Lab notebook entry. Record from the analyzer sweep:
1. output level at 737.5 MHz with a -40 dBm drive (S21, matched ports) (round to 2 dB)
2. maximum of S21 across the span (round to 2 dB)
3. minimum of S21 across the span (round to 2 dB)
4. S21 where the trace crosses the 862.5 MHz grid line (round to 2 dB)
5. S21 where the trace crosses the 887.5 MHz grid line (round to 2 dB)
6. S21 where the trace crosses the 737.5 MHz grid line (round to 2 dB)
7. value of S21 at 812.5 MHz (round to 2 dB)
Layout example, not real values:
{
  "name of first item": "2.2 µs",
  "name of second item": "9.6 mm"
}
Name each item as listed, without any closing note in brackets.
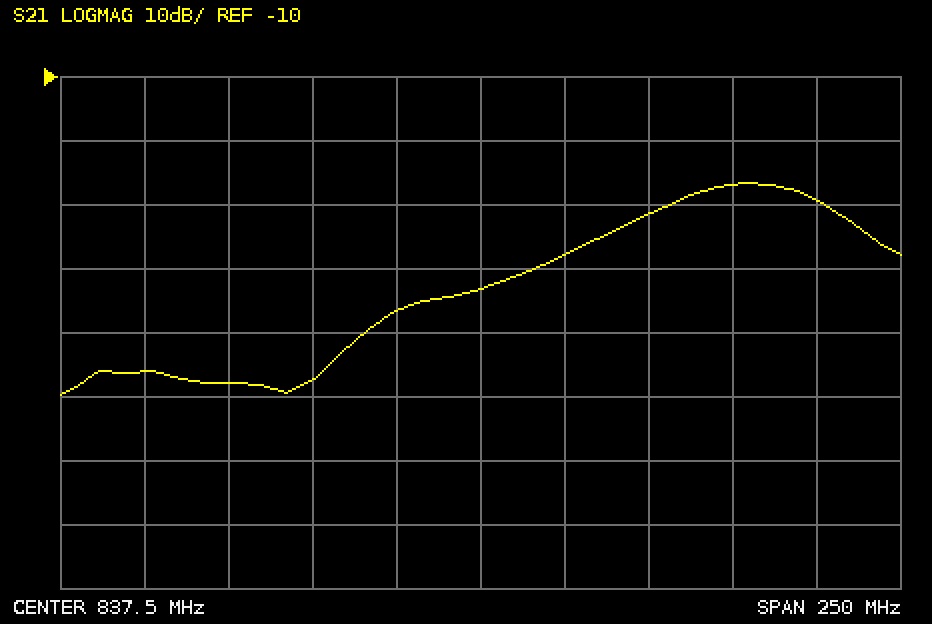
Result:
{
  "output level at 737.5 MHz with a -40 dBm drive (S21, matched ports)": "-96 dBm",
  "maximum of S21 across the span": "-26 dB",
  "minimum of S21 across the span": "-60 dB",
  "S21 where the trace crosses the 862.5 MHz grid line": "-38 dB",
  "S21 where the trace crosses the 887.5 MHz grid line": "-32 dB",
  "S21 where the trace crosses the 737.5 MHz grid line": "-56 dB",
  "value of S21 at 812.5 MHz": "-46 dB"
}
